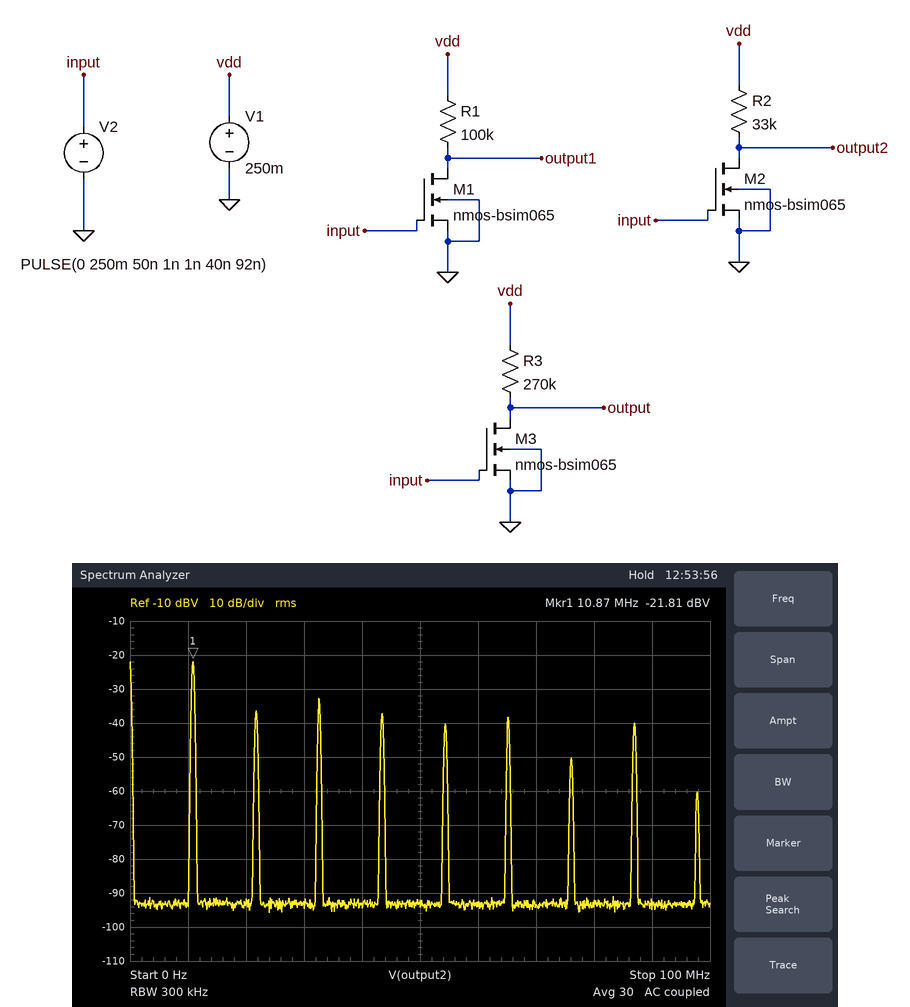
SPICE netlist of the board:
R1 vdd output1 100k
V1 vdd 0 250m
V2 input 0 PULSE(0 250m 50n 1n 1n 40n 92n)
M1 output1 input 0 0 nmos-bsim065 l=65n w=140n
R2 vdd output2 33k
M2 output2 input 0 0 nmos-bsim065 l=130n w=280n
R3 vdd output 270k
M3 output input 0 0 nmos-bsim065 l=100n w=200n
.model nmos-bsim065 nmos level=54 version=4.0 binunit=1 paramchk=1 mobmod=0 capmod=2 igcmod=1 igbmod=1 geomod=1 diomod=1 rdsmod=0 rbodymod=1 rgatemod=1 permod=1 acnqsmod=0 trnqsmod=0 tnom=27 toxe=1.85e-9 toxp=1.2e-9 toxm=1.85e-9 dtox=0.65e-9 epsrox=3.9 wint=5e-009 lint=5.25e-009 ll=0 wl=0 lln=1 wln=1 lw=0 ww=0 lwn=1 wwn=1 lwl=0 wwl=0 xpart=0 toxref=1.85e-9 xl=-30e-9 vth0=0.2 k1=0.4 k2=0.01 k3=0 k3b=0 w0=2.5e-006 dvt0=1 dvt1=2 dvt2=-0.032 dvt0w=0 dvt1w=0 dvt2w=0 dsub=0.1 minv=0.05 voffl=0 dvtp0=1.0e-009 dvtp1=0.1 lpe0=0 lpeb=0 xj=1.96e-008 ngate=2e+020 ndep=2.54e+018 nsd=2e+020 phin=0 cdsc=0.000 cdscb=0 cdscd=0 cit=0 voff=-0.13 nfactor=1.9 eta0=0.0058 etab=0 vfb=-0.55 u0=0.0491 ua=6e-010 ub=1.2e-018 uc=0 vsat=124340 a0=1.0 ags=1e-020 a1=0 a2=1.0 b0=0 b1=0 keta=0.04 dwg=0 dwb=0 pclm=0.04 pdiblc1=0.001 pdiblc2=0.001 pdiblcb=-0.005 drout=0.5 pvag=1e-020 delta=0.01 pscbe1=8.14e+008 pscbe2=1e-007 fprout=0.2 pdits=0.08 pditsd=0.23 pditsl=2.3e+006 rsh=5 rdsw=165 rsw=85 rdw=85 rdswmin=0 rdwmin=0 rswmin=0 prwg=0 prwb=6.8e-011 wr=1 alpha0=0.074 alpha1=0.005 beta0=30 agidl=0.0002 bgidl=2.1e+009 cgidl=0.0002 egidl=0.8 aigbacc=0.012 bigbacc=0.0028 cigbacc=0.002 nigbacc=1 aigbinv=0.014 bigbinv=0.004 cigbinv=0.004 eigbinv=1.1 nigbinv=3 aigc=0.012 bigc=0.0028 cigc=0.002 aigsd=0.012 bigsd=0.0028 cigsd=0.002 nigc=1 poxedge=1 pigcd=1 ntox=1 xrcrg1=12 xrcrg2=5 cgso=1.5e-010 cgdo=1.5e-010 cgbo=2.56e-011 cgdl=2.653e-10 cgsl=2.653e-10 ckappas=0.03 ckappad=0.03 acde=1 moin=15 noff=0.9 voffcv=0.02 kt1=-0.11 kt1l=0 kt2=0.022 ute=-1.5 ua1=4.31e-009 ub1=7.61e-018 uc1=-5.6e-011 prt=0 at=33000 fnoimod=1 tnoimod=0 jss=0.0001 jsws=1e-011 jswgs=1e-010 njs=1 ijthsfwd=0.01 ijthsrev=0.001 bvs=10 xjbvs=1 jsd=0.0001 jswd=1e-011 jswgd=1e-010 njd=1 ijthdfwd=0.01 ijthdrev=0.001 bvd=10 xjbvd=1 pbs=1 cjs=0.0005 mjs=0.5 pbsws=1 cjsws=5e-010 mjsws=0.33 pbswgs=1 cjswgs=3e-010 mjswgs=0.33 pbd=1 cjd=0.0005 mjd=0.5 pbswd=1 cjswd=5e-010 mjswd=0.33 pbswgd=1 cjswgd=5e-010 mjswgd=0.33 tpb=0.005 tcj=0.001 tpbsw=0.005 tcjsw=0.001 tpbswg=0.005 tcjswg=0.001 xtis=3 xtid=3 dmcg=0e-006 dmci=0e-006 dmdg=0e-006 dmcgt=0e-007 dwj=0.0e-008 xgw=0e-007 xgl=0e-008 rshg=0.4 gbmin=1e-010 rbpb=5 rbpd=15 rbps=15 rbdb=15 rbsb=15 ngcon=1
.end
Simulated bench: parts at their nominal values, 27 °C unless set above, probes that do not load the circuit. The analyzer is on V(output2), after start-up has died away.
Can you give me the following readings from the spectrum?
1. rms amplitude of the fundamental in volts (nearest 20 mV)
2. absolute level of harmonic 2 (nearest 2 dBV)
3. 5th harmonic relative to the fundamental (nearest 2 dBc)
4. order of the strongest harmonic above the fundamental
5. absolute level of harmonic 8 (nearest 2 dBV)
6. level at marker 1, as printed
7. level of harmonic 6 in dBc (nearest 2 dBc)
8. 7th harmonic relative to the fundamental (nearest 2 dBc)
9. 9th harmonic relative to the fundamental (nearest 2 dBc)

80 mV
-36 dBV
-18 dBc
3
-40 dBV
-21.81 dBV
-16 dBc
-28 dBc
-38 dBc
